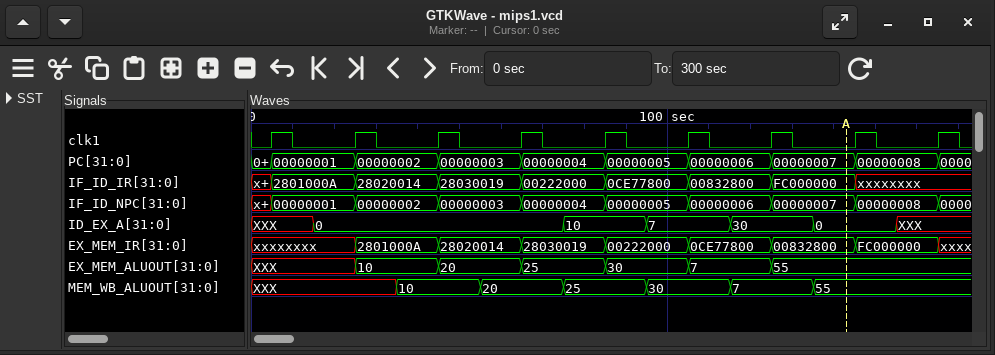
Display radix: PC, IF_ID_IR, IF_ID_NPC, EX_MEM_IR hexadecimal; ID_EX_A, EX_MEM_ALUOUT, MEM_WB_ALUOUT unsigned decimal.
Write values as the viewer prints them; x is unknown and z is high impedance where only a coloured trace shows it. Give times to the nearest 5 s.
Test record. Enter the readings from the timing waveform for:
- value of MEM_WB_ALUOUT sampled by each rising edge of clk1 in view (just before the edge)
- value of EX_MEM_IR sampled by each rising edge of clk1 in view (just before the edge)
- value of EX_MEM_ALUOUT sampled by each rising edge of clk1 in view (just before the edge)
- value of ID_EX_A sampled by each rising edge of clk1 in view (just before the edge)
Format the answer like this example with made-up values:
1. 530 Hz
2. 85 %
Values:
1. XXX, XXX, 10, 20, 25, 30, 7, 55, 55
2. xxxxxxxx, xxxxxxxx, 2801000A, 28020014, 28030019, 00222000, 0CE77800, 00832800, FC000000
3. XXX, XXX, 10, 20, 25, 30, 7, 55, 55
4. XXX, 0, 0, 0, 10, 7, 30, 0, XXX
